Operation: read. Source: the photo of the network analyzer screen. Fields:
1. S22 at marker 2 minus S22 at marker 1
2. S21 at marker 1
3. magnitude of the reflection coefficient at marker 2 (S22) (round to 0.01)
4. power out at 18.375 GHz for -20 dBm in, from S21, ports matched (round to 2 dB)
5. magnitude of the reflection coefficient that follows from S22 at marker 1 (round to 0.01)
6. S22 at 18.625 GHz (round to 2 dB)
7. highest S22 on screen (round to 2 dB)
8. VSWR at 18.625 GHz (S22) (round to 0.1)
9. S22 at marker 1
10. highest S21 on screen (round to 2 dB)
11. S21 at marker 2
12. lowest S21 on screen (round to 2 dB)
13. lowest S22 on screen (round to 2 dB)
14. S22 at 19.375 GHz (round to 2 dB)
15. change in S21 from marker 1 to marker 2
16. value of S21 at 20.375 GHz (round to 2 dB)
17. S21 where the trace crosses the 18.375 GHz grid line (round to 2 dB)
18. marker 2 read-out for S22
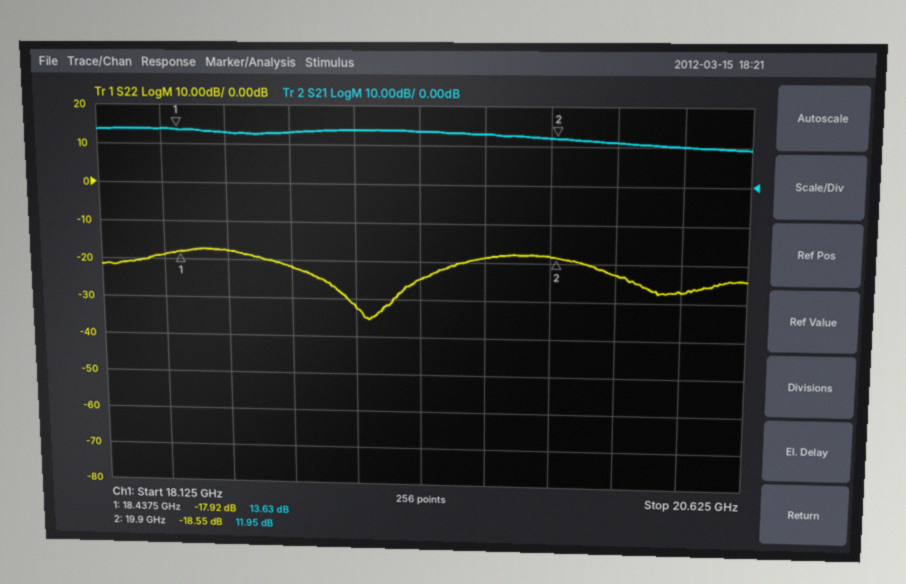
-0.63 dB
13.63 dB
0.12
-6 dBm
0.13
-18 dB
-18 dB
1.3
-17.92 dB
14 dB
11.95 dB
10 dB
-36 dB
-24 dB
-1.68 dB
10 dB
14 dB
-18.55 dB
